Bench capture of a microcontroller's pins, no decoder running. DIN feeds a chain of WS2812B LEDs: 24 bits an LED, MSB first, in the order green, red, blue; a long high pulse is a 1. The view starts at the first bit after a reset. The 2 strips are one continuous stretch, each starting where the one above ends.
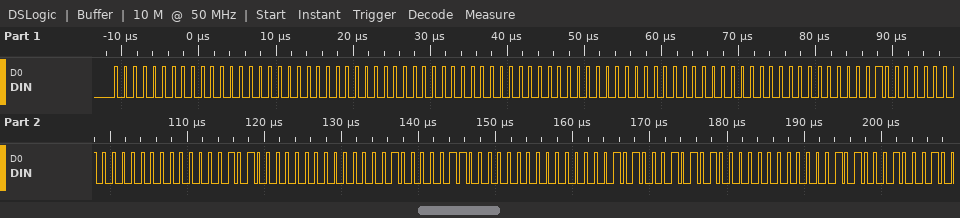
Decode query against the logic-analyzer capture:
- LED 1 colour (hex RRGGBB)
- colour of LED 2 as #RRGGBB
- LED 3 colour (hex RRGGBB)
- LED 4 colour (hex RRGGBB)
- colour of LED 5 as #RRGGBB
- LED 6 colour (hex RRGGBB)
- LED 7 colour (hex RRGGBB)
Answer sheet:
#000000
#000000
#000000
#000100
#000502
#000C05
#00150A
